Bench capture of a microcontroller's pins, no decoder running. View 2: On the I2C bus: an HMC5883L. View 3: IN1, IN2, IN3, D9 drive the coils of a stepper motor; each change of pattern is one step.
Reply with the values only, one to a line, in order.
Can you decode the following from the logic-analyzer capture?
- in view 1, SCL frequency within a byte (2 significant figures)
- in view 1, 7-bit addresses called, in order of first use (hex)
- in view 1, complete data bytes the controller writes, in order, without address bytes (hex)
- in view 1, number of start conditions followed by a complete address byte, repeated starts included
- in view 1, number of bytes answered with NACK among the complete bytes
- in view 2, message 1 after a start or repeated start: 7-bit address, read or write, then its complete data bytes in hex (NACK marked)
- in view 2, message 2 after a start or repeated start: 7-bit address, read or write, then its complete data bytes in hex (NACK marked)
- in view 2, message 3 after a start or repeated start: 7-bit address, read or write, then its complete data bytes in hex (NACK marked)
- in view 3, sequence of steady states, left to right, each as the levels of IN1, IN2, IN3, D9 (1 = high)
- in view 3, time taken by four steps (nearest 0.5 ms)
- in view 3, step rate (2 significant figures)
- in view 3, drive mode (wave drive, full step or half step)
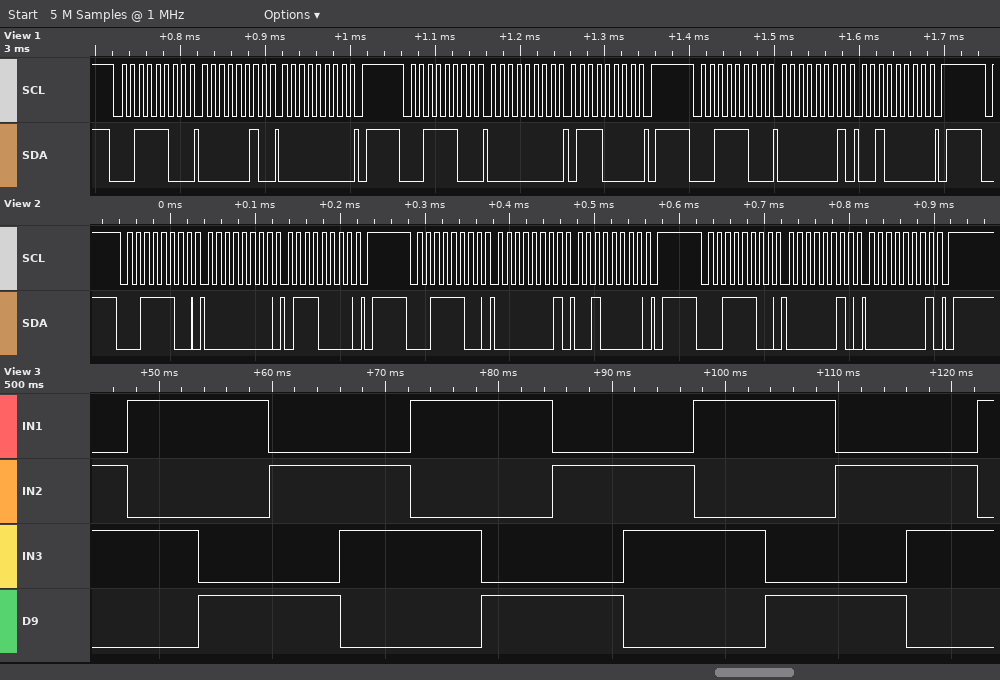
100 kHz
0x1E
02 00 00 70 01 20
3
0
0x1E write: 00 70
0x1E write: 01 20
0x1E write: 02 01
0110 1010 1001 0101 0110 1010 1001 0101 0110 1010 1001 0101 0110 1010
25.0 ms
160 steps/s
full step
